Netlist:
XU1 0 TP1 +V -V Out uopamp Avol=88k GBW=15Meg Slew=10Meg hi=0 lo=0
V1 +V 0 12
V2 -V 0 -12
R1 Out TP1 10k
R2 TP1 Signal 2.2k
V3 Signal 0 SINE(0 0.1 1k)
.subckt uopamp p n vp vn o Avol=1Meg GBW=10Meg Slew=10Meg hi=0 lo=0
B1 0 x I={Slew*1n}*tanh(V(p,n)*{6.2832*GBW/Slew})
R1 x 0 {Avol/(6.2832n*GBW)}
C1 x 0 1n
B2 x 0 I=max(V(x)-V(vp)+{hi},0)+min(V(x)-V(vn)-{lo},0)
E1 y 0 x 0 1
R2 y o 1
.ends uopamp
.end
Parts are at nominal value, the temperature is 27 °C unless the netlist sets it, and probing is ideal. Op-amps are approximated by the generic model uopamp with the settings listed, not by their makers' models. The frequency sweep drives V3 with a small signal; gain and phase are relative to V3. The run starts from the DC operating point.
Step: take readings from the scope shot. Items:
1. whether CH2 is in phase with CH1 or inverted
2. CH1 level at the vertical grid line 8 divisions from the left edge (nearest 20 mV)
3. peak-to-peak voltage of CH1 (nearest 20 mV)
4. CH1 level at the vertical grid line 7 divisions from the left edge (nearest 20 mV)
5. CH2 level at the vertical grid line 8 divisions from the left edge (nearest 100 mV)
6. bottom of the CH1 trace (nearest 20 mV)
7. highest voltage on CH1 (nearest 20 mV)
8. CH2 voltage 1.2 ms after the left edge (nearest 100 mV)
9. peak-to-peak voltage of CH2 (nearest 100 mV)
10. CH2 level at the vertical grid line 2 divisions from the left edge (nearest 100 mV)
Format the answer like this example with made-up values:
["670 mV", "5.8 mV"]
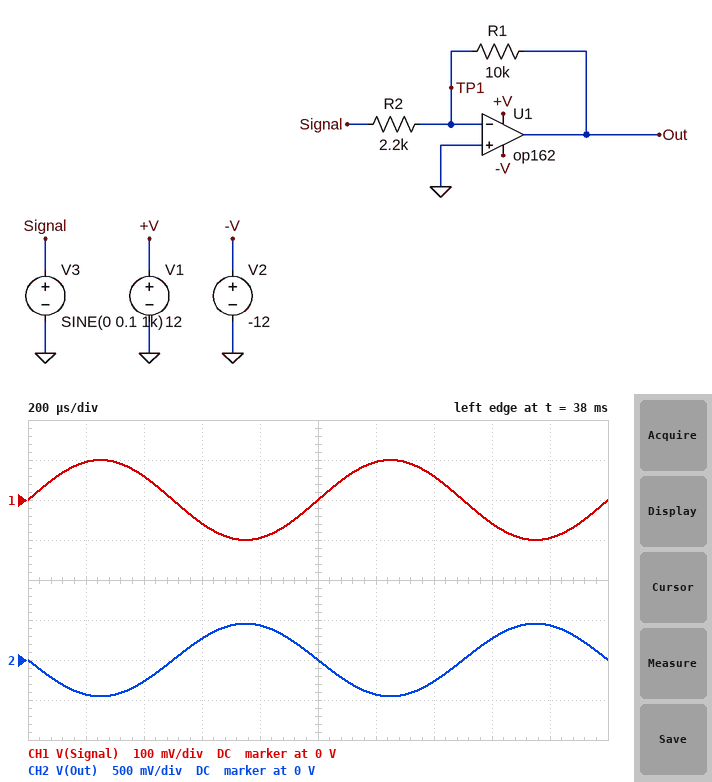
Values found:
["inverted", "-60 mV", "200 mV", "60 mV", "300 mV", "-100 mV", "100 mV", "-400 mV", "900 mV", "-300 mV"]
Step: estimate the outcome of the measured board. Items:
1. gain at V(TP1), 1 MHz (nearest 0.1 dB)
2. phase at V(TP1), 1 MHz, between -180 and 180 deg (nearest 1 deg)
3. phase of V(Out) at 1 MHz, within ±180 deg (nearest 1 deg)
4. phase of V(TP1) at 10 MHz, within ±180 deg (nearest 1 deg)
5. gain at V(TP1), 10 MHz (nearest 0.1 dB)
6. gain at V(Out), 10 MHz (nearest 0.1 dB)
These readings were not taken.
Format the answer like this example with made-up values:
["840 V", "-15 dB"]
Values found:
["-10.9 dB", "70 deg", "160 deg", "15 deg", "-2.0 dB", "1.5 dB"]
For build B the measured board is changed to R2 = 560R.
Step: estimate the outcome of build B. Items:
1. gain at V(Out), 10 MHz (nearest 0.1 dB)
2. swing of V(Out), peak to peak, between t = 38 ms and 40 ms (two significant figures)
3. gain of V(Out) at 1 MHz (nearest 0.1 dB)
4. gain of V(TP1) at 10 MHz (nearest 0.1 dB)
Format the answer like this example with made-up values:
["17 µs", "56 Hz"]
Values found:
["3.0 dB", "3.6 V", "20.9 dB", "-0.5 dB"]
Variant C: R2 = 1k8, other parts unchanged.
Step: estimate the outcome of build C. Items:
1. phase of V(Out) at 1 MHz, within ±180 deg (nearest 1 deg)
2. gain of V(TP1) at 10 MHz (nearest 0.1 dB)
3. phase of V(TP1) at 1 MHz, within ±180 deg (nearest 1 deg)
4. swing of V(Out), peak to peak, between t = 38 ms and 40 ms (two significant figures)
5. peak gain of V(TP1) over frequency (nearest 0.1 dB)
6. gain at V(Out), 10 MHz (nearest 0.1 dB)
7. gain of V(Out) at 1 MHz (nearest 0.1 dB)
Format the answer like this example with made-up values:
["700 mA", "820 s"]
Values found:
["156 deg", "-1.7 dB", "66 deg", "1.1 V", "-1.4 dB", "1.9 dB", "14.1 dB"]
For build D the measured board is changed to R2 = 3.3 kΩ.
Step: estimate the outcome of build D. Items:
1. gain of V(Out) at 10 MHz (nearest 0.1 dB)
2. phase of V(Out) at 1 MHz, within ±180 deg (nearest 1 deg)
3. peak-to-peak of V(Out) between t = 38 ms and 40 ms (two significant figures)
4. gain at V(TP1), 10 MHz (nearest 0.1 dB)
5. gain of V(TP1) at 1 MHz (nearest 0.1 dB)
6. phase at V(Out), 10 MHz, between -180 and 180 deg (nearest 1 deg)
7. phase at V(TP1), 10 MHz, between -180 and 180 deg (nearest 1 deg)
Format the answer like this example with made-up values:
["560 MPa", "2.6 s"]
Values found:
["0.5 dB", "165 deg", "610 mV", "-3.0 dB", "-14.2 dB", "110 deg", "20 deg"]
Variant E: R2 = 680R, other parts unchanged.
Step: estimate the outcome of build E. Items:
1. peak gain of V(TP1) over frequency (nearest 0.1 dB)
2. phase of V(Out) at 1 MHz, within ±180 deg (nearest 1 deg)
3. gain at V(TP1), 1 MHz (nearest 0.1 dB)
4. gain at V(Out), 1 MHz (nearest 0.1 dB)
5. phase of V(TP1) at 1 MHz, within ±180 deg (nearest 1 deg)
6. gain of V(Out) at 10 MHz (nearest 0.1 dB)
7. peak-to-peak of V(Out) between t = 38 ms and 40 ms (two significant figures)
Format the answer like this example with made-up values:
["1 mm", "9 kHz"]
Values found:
["-0.6 dB", "134 deg", "-3.4 dB", "20.1 dB", "44 deg", "2.9 dB", "2.9 V"]
